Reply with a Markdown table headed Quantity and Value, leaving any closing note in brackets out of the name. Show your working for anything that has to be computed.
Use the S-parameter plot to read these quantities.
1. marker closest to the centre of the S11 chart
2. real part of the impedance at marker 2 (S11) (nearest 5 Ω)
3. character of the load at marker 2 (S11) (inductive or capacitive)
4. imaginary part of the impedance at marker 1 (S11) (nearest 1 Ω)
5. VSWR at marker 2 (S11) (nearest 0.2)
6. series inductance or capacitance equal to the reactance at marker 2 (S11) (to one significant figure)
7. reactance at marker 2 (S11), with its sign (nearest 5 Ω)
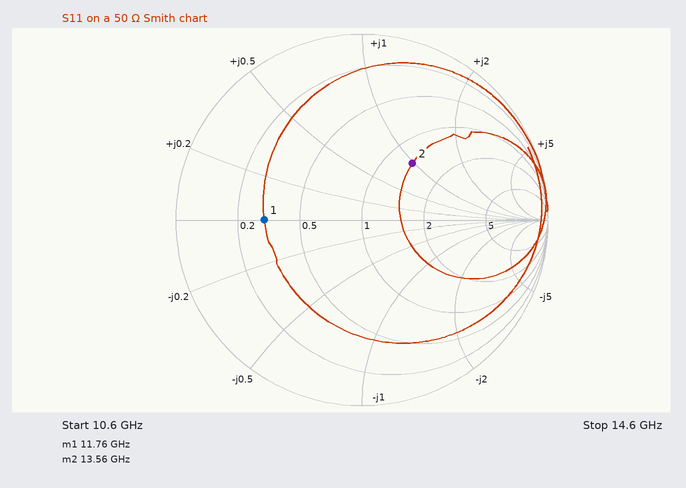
| Quantity | Value |
|---|---|
| marker closest to the centre of the S11 chart | marker 2 |
| real part of the impedance at marker 2 (S11) | 65 Ω |
| character of the load at marker 2 (S11) | inductive |
| imaginary part of the impedance at marker 1 (S11) | 0 Ω |
| VSWR at marker 2 (S11) | 2.4 |
| series inductance or capacitance equal to the reactance at marker 2 (S11) | L = 50 Ω/(2π × 13.56 GHz) ≈ 587 pH, so 600 pH to one significant figure |
| reactance at marker 2 (S11), with its sign | +50 Ω |
